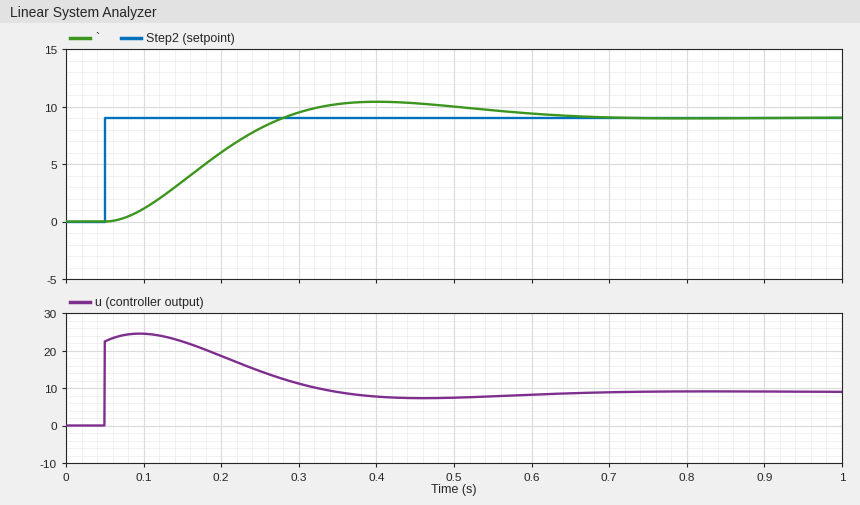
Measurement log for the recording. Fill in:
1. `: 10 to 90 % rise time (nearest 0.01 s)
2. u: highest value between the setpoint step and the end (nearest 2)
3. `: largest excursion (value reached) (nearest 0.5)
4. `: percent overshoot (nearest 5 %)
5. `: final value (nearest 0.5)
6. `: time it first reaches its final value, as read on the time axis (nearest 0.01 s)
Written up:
0.16 s
24
10.5
15 %
9.0
0.28 s
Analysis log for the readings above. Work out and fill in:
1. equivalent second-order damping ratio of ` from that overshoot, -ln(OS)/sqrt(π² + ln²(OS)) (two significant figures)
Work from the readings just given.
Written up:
0.52
